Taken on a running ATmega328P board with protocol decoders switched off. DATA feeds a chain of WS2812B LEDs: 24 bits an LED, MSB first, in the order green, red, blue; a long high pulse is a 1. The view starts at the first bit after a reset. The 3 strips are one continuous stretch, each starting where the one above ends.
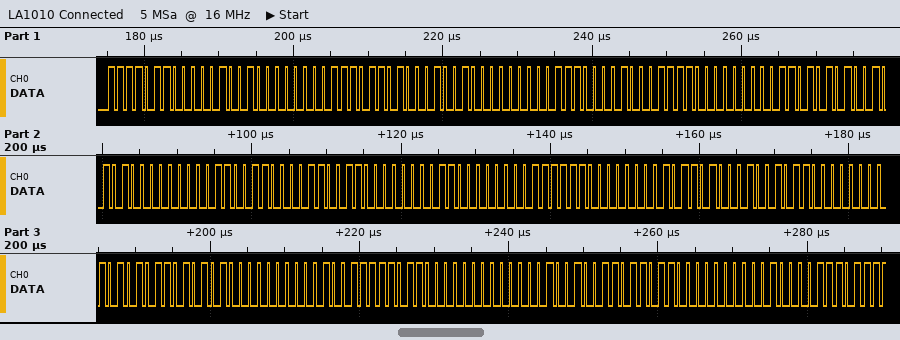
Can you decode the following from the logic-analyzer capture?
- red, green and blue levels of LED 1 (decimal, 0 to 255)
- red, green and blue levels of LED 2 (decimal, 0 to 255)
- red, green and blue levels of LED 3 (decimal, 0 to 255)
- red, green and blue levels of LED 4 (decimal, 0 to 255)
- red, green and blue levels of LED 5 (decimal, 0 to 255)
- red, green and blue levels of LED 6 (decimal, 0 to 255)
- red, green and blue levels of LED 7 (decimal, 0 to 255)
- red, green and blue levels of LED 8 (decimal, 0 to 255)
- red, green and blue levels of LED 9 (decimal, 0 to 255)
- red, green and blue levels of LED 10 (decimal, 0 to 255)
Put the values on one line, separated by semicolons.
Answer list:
9, 246, 0; 18, 237, 0; 30, 225, 0; 42, 213, 0; 51, 204, 0; 63, 192, 0; 75, 180, 0; 84, 171, 0; 96, 159, 0; 108, 147, 0
